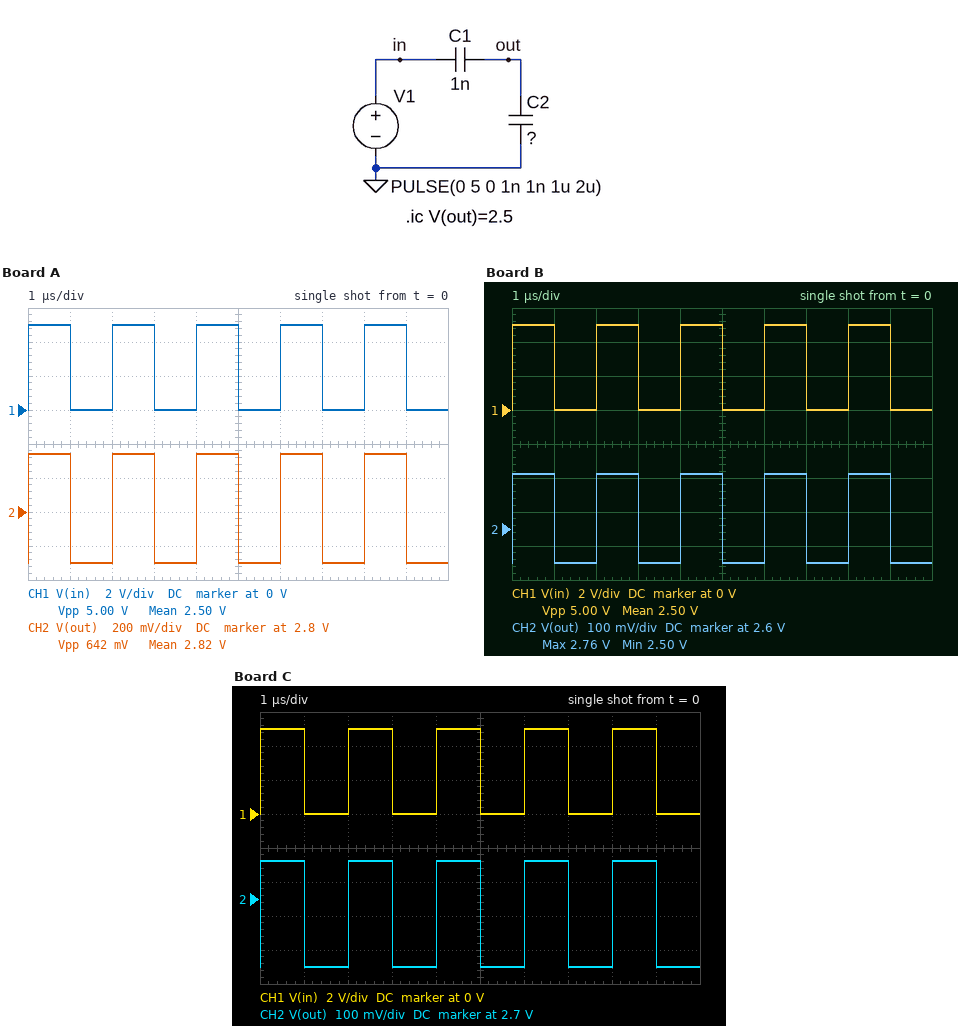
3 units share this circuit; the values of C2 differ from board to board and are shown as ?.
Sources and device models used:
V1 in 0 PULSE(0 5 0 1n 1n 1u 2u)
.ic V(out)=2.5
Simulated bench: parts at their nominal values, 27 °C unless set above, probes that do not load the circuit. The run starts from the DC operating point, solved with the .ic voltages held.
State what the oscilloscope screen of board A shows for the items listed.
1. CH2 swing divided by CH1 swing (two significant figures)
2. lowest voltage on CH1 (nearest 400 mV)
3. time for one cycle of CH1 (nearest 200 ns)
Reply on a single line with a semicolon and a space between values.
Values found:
0.13; 0 V; 2.0 µs
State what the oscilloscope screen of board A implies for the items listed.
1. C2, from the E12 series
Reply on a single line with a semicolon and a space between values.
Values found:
6.8 nF
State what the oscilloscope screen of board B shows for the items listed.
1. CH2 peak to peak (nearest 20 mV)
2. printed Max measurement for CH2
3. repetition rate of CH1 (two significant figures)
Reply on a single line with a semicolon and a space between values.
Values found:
260 mV; 2.76 V; 500 kHz
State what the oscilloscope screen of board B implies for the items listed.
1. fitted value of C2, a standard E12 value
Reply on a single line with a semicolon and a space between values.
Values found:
18 nF
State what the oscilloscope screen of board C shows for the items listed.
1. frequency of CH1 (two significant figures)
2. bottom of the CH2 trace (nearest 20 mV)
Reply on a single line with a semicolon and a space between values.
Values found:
500 kHz; 2.50 V
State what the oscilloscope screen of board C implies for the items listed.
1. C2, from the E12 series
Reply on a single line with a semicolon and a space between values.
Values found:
15 nF
